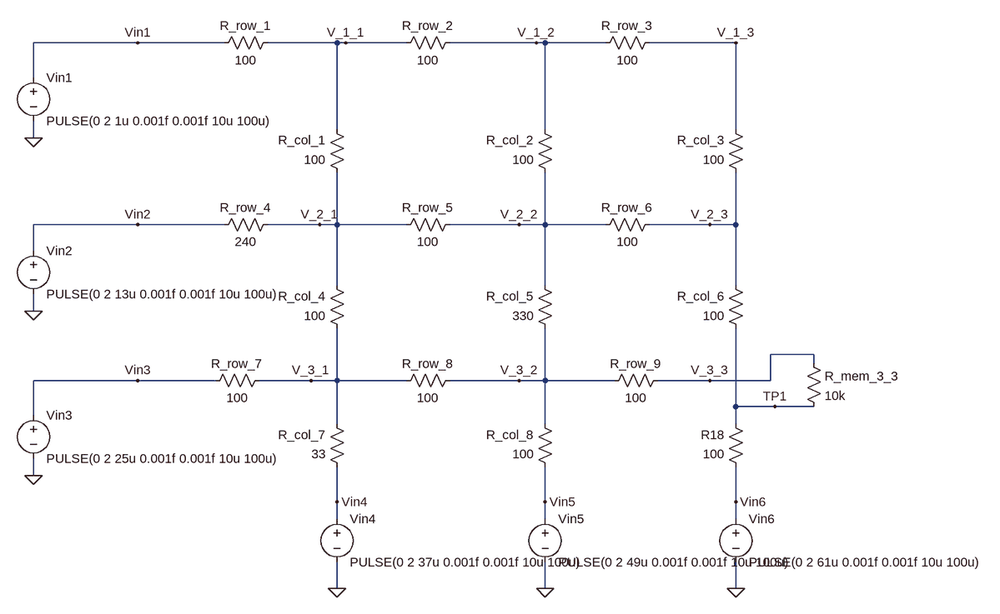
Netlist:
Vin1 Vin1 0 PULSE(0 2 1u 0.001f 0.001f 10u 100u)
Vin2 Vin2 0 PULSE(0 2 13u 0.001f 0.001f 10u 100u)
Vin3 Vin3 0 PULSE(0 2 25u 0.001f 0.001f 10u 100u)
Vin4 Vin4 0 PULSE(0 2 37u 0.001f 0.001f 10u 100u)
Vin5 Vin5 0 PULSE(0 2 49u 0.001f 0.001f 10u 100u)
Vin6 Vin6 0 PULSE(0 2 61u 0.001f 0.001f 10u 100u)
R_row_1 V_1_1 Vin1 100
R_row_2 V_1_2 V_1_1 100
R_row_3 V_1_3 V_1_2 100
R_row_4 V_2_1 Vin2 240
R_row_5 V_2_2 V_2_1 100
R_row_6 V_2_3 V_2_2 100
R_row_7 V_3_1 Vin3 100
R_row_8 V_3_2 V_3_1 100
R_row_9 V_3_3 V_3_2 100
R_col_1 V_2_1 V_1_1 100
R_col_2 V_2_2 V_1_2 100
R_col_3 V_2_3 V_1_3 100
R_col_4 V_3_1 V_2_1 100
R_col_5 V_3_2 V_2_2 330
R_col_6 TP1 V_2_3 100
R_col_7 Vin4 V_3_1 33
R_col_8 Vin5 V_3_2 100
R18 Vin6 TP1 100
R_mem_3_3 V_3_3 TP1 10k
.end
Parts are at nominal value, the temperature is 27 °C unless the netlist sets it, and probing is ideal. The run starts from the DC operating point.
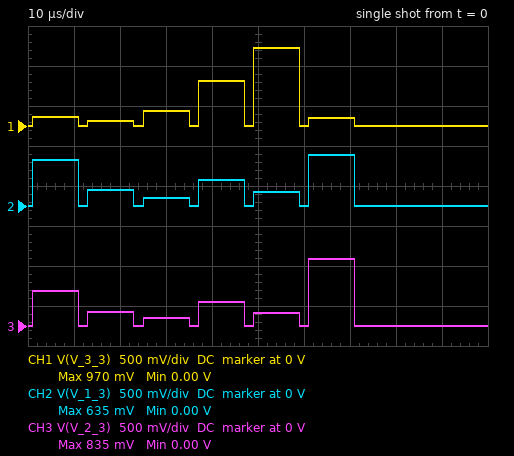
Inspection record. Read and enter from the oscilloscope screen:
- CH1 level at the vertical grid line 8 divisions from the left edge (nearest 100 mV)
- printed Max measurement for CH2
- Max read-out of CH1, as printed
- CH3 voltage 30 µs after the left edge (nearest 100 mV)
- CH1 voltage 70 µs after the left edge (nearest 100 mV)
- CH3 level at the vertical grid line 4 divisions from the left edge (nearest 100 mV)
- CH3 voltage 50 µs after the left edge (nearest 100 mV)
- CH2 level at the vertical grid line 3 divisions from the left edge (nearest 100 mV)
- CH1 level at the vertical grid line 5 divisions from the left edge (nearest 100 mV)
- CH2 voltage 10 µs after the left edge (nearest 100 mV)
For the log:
0 V
635 mV
970 mV
100 mV
100 mV
300 mV
200 mV
100 mV
1.0 V
600 mV
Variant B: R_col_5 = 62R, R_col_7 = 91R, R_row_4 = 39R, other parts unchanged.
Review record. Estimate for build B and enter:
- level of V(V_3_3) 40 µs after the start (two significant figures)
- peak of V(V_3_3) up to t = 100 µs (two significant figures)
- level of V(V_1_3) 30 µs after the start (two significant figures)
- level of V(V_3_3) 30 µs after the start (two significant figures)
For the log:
260 mV
810 mV
120 mV
230 mV
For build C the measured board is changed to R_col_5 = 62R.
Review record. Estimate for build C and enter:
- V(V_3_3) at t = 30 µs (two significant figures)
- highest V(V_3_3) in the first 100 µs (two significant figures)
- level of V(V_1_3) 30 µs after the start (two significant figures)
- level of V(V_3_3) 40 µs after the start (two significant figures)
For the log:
180 mV
810 mV
120 mV
530 mV
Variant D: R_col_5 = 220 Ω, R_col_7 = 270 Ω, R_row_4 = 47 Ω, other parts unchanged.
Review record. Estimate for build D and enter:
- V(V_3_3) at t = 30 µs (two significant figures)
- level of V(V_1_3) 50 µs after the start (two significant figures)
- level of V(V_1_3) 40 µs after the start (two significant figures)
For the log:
340 mV
200 mV
51 mV
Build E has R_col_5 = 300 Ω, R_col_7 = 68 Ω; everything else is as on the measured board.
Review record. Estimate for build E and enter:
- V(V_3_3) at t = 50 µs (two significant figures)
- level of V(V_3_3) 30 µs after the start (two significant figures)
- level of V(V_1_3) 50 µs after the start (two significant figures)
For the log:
1.0 V
270 mV
200 mV
